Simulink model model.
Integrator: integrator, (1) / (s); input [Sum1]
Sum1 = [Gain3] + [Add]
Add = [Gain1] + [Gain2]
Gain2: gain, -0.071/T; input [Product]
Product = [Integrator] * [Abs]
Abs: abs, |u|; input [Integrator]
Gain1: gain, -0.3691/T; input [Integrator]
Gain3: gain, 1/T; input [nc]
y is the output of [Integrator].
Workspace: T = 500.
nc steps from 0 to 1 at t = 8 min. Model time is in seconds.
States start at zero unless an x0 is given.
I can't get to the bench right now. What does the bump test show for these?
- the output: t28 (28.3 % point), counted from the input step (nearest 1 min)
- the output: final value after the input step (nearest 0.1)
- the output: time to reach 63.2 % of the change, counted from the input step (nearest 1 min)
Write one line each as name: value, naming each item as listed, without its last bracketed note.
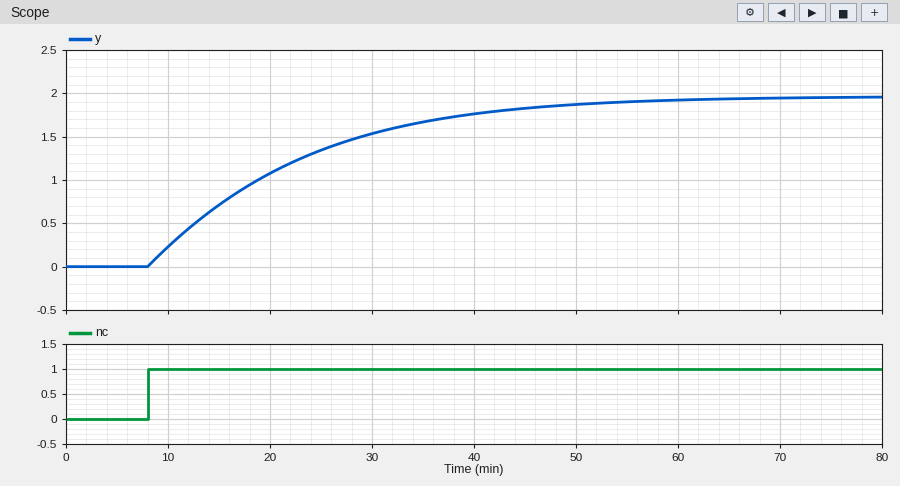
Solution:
the output: t28 (28.3 % point), counted from the input step: 5 min
the output: final value after the input step: 2.0
the output: time to reach 63.2 % of the change, counted from the input step: 15 min
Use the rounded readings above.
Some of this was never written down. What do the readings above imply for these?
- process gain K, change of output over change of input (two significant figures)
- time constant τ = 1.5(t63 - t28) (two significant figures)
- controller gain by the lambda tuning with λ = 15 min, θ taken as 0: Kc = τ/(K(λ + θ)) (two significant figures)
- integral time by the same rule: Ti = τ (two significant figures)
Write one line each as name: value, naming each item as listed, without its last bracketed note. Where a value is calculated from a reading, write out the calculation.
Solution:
process gain K, change of output over change of input: (2 - 0) / 1 = 2.0
time constant τ = 1.5(t63 - t28): 1.5 × (15 - 5) = 15 min
controller gain by the lambda tuning with λ = 15 min, θ taken as 0: Kc = τ/(K(λ + θ)): 15 / (2 × (15 + 0)) = 0.50
integral time by the same rule: Ti = τ: 15 min
